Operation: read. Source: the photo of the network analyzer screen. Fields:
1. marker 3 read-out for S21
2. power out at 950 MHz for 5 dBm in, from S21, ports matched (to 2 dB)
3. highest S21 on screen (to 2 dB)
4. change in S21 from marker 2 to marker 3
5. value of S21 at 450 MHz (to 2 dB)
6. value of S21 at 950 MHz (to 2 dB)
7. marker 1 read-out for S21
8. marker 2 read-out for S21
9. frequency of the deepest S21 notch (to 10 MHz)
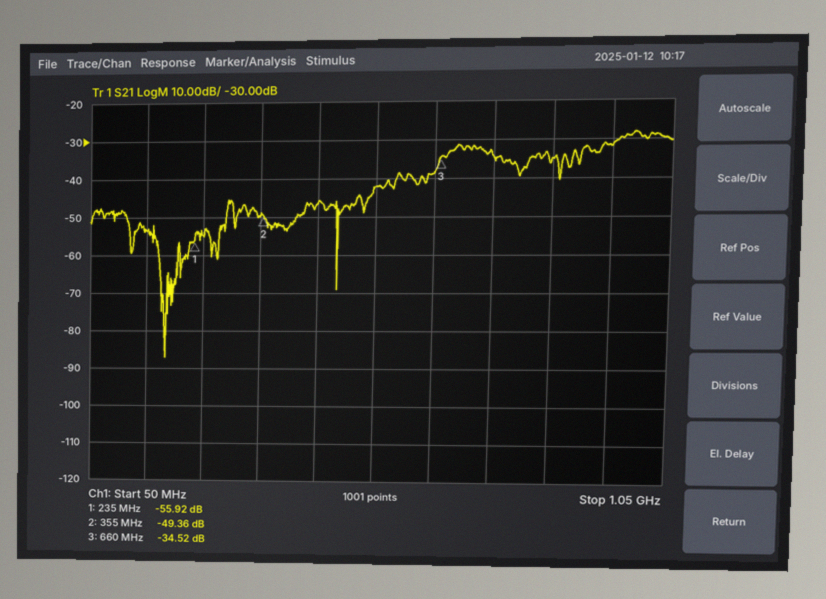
-34.52 dB
-26 dBm
-28 dB
14.84 dB
-46 dB
-32 dB
-55.92 dB
-49.36 dB
180 MHz
